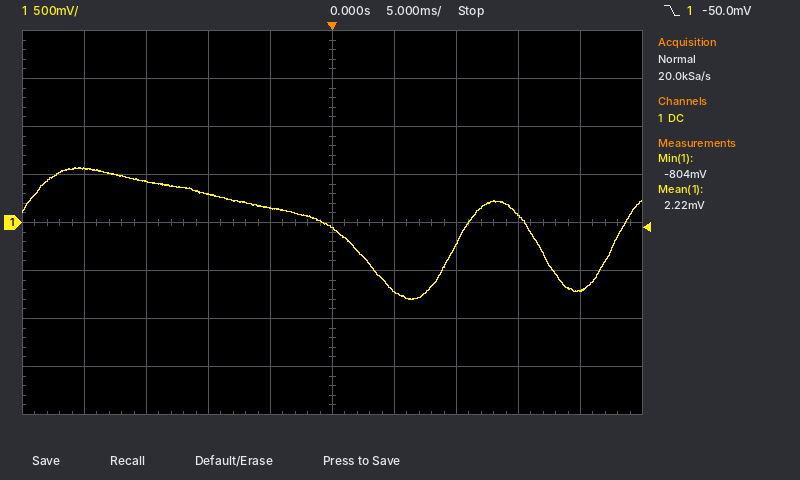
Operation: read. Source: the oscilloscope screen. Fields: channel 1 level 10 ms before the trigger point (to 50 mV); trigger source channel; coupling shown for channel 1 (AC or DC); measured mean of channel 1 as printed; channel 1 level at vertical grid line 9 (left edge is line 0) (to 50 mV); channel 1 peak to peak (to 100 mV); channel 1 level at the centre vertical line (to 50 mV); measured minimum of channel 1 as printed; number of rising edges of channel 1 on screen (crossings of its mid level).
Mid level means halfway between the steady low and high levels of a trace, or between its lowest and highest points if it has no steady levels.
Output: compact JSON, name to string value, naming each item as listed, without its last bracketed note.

{"channel 1 level 10 ms before the trigger point": "300 mV", "trigger source channel": "channel 1", "coupling shown for channel 1": "DC", "measured mean of channel 1 as printed": "2.22 mV", "channel 1 level at vertical grid line 9 (left edge is line 0)": "-700 mV", "channel 1 peak to peak": "1.40 V", "channel 1 level at the centre vertical line": "-50 mV", "measured minimum of channel 1 as printed": "-804 mV", "number of rising edges of channel 1 on screen": "2"}
